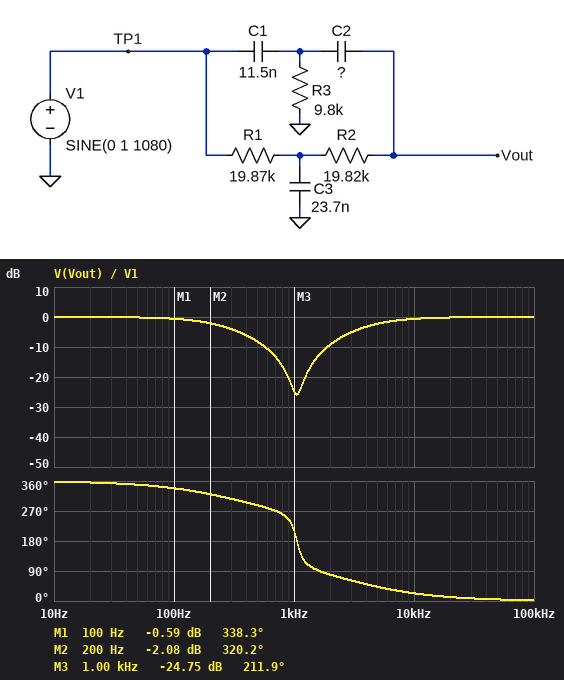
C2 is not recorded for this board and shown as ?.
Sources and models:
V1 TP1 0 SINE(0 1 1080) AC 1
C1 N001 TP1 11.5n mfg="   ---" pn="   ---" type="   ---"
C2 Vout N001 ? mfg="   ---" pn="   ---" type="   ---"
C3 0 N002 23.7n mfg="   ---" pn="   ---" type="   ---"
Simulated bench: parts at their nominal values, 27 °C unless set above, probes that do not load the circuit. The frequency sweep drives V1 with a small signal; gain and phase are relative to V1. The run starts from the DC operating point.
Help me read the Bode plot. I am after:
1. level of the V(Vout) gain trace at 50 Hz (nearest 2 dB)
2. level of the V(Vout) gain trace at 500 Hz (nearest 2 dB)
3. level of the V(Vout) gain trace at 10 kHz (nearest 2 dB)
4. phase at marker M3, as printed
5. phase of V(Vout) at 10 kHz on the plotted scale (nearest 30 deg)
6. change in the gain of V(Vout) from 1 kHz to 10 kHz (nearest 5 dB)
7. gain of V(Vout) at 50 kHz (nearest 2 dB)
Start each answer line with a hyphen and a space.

- 0 dB
- -8 dB
- 0 dB
- 211.9 deg
- 30 deg
- 25 dB
- 0 dB
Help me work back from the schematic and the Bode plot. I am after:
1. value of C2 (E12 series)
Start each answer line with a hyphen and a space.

- 3.9 nF
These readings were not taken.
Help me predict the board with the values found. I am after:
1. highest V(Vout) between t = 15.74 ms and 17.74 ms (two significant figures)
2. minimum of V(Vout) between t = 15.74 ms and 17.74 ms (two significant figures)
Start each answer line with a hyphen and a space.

- 52 mV
- -52 mV
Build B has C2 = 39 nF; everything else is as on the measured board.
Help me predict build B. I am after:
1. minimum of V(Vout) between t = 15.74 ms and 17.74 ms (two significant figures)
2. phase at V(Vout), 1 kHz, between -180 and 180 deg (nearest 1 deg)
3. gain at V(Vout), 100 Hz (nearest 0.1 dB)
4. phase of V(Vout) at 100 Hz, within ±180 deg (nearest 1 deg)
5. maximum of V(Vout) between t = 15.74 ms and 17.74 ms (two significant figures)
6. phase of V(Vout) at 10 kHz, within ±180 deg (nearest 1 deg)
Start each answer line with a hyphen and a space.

- -340 mV
- 61 deg
- -4.9 dB
- -48 deg
- 340 mV
- 13 deg
